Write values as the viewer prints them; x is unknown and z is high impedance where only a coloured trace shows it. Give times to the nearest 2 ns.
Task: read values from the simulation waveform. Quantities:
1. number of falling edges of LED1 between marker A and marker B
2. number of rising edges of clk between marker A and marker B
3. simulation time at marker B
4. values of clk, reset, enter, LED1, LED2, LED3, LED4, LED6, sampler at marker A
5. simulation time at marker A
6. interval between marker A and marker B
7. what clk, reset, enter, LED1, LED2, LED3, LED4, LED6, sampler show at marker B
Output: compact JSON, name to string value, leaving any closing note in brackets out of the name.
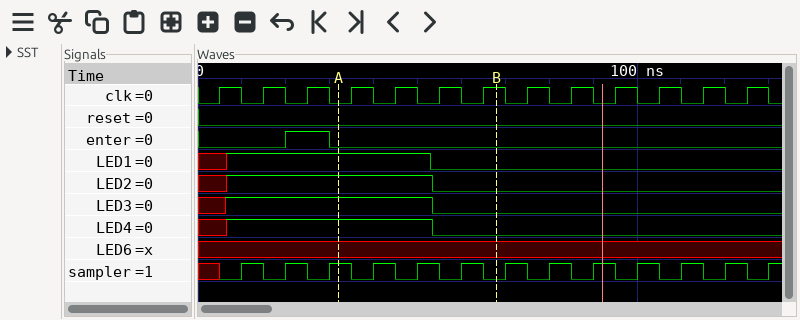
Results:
{"number of falling edges of LED1 between marker A and marker B": "1", "number of rising edges of clk between marker A and marker B": "4", "simulation time at marker B": "68 ns", "values of clk, reset, enter, LED1, LED2, LED3, LED4, LED6, sampler at marker A": "clk=0, reset=0, enter=0, LED1=1, LED2=1, LED3=1, LED4=1, LED6=x, sampler=1", "simulation time at marker A": "32 ns", "interval between marker A and marker B": "36 ns", "what clk, reset, enter, LED1, LED2, LED3, LED4, LED6, sampler show at marker B": "clk=1, reset=0, enter=0, LED1=0, LED2=0, LED3=0, LED4=0, LED6=x, sampler=0"}
